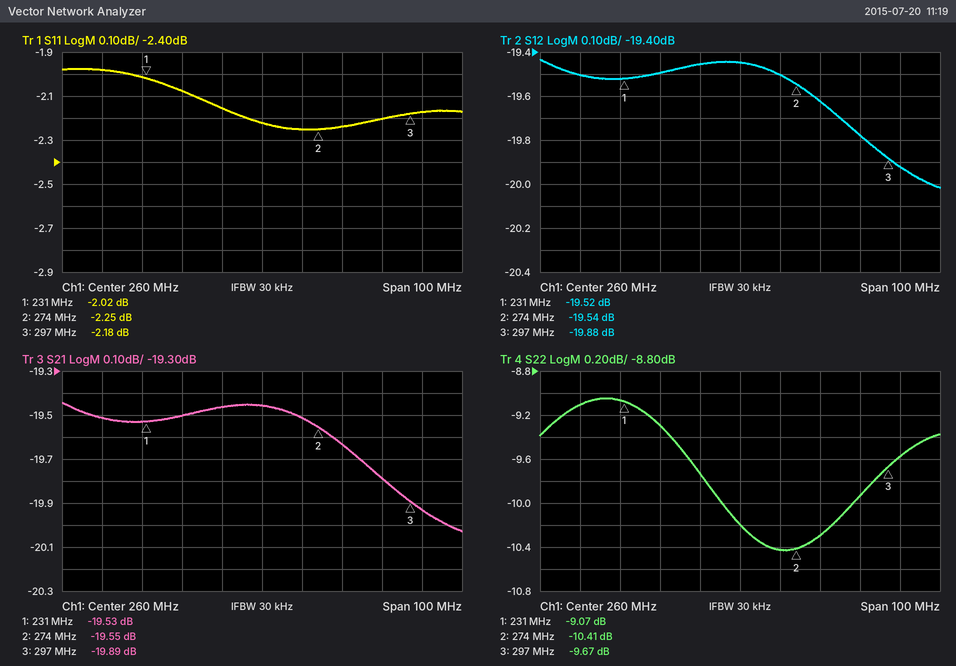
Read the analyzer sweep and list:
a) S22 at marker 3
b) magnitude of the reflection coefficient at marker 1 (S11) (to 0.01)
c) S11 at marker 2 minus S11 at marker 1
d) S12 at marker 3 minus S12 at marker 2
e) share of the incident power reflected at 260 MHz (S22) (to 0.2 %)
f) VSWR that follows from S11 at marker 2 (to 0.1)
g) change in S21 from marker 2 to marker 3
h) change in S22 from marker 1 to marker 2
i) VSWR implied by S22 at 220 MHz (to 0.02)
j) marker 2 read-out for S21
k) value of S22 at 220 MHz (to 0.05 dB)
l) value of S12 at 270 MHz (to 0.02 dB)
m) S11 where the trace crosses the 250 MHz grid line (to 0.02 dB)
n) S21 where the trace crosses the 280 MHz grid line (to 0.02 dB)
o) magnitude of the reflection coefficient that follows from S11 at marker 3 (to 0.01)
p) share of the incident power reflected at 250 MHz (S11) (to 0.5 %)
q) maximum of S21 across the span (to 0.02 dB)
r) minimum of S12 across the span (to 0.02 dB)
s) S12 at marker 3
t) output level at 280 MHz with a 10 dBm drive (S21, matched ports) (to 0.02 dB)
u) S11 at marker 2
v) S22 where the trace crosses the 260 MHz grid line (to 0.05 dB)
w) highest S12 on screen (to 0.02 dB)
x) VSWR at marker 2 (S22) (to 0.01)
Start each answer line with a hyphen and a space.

- -9.67 dB
- 0.79
- -0.23 dB
- -0.34 dB
- 9.6 %
- 7.8
- -0.34 dB
- -1.34 dB
- 2.08
- -19.55 dB
- -9.10 dB
- -19.50 dB
- -2.16 dB
- -19.64 dB
- 0.78
- 61.0 %
- -19.44 dB
- -20.02 dB
- -19.88 dB
- -9.64 dBm
- -2.25 dB
- -10.20 dB
- -19.44 dB
- 1.86
